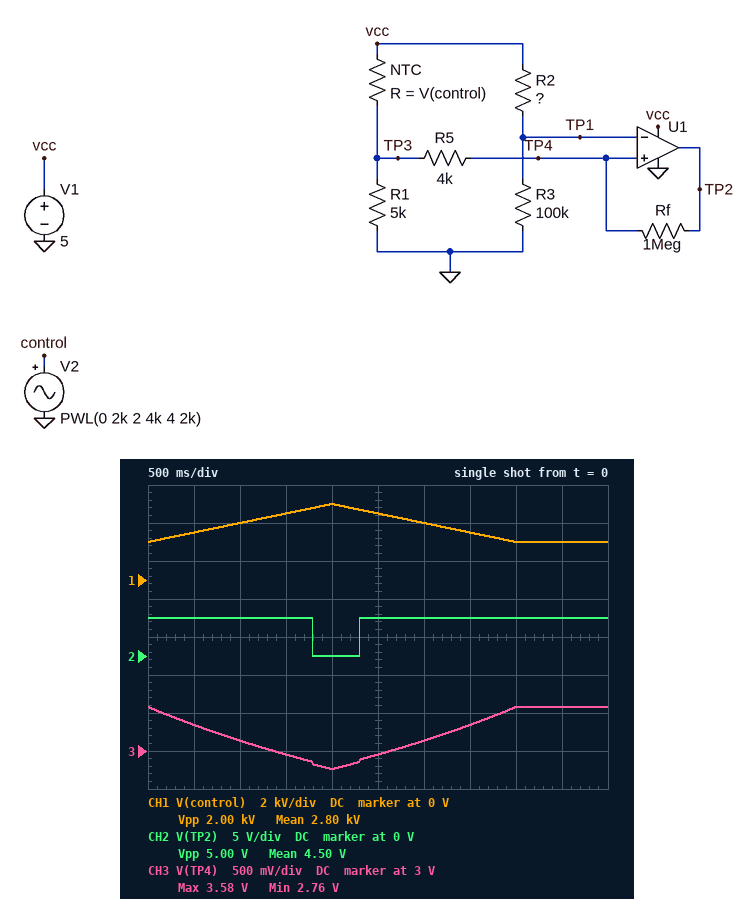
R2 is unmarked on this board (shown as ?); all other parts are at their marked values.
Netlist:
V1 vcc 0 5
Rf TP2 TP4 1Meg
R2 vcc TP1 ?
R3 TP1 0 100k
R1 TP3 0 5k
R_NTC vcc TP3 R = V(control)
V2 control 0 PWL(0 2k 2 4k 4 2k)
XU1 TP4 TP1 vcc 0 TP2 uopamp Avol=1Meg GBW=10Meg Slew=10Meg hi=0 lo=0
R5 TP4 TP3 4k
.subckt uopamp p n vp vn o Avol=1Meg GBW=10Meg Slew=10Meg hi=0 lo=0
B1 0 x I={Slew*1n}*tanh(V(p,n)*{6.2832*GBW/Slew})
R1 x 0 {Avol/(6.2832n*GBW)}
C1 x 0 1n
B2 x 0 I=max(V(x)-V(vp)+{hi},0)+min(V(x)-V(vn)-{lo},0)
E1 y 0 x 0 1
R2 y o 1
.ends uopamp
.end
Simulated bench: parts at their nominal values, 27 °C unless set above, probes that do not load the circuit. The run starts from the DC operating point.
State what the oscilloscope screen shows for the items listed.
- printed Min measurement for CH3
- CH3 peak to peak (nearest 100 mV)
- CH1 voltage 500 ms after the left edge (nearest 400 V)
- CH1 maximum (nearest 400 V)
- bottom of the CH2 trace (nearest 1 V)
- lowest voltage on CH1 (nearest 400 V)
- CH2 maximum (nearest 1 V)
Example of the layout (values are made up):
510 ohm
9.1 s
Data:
2.76 V
800 mV
2.4 kV
4.0 kV
0 V
2.0 kV
5 V
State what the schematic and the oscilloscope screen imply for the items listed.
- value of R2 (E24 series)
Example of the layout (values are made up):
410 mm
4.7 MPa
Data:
75 kΩ
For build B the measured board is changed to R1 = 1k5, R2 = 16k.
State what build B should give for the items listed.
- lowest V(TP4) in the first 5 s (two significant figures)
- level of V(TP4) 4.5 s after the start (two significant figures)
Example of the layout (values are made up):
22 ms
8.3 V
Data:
1.4 V
2.1 V
